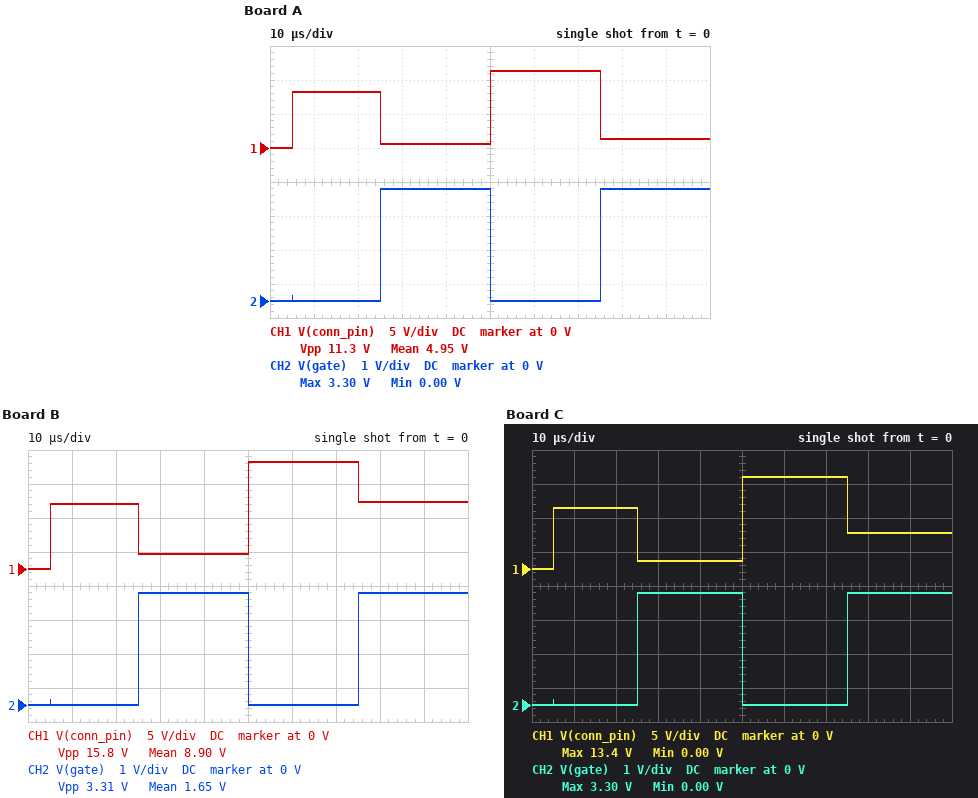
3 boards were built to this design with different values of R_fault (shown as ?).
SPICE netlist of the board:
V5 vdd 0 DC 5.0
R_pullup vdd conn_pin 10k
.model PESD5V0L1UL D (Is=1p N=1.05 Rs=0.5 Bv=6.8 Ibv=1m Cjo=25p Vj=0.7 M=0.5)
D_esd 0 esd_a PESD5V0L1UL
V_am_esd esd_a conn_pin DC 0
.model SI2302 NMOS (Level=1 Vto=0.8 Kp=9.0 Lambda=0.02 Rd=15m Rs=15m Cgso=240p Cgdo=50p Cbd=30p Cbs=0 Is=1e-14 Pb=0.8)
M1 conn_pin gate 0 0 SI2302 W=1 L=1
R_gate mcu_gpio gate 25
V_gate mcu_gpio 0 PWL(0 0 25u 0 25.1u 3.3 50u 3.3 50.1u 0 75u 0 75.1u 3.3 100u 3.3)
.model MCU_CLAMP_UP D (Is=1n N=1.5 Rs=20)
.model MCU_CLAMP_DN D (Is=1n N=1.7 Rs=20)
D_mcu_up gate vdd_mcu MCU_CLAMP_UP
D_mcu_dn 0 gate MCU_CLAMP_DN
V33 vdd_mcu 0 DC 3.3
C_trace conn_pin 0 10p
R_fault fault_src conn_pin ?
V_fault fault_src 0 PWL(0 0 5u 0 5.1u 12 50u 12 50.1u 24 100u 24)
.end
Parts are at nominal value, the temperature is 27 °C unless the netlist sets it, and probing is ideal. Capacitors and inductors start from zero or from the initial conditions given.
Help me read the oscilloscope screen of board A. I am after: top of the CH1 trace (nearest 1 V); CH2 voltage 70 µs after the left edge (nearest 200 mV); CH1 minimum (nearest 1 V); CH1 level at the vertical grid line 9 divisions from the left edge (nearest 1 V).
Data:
11 V
0 V
0 V
1 V
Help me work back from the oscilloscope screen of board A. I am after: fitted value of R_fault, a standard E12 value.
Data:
1.5 Ω
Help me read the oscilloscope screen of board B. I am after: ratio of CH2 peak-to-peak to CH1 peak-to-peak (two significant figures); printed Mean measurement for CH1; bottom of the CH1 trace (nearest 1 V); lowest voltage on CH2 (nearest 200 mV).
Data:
0.21
8.90 V
0 V
0 V
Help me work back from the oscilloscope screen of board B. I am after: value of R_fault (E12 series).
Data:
0.47 Ω
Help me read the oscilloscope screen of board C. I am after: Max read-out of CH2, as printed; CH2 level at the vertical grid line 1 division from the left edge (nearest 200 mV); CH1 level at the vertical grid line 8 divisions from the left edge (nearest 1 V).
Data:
3.30 V
0 V
5 V
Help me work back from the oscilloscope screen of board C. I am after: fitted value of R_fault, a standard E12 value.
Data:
0.82 Ω
